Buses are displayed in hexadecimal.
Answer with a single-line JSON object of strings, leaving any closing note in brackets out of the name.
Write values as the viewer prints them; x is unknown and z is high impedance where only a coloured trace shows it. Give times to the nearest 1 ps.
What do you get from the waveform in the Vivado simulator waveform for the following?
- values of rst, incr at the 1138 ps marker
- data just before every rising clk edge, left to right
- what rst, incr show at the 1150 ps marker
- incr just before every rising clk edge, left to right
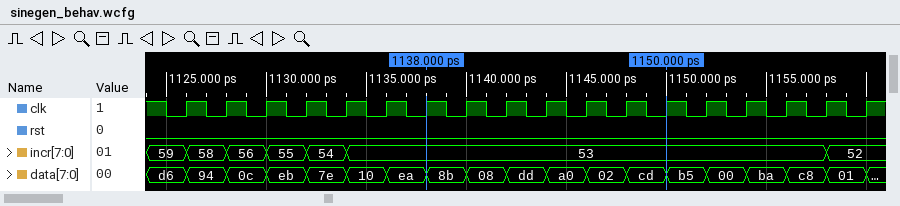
{"values of rst, incr at the 1138 ps marker": "rst=0, incr=53", "data just before every rising clk edge, left to right": "d6, 94, 0c, eb, 7e, 10, ea, 8b, 08, dd, a0, 02, cd, b5, 00, ba, c8, 01", "what rst, incr show at the 1150 ps marker": "rst=0, incr=53", "incr just before every rising clk edge, left to right": "59, 58, 56, 55, 54, 53, 53, 53, 53, 53, 53, 53, 53, 53, 53, 53, 53, 52"}
